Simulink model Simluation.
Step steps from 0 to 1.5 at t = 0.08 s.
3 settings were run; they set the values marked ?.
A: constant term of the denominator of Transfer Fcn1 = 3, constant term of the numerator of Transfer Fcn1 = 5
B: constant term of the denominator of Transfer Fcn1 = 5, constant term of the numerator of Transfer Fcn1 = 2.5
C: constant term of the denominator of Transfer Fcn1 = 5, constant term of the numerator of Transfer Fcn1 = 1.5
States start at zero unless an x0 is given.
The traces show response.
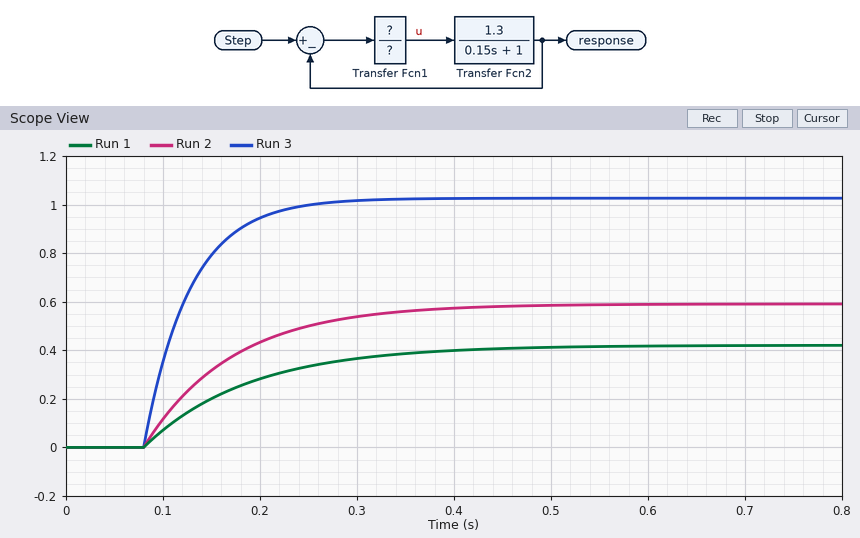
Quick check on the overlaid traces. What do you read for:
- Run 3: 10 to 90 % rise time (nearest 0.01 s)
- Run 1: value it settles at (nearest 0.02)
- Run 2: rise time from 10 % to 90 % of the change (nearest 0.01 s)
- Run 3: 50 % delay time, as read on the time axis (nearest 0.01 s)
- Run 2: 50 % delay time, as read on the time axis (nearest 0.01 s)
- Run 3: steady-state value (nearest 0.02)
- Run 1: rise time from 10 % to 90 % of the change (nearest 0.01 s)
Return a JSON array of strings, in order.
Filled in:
["0.10 s", "0.42", "0.20 s", "0.11 s", "0.14 s", "1.02", "0.24 s"]
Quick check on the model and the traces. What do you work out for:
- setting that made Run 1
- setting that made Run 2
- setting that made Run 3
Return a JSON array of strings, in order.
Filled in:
["C", "B", "A"]
